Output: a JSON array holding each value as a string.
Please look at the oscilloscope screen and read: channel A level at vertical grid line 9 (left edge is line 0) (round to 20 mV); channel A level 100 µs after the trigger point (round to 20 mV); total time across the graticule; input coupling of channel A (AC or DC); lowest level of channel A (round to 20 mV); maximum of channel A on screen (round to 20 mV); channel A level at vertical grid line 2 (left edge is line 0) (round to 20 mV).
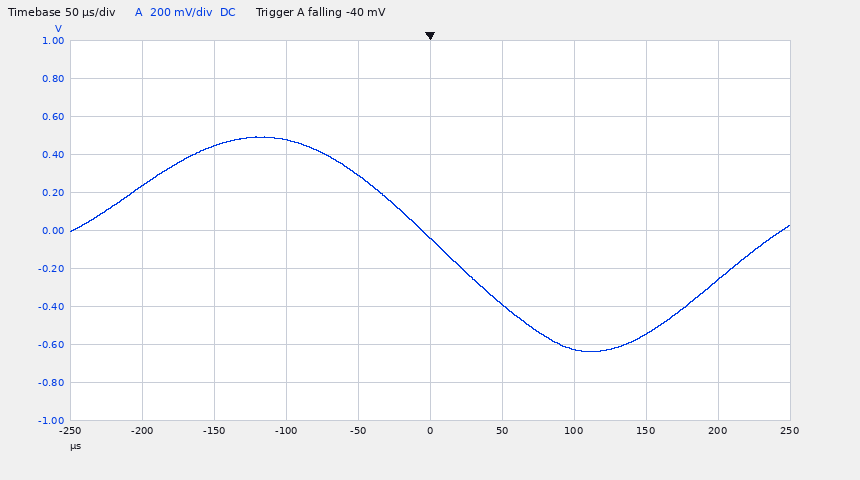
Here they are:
["-260 mV", "-620 mV", "500 µs", "DC", "-640 mV", "500 mV", "440 mV"]
